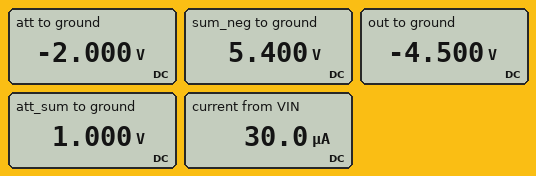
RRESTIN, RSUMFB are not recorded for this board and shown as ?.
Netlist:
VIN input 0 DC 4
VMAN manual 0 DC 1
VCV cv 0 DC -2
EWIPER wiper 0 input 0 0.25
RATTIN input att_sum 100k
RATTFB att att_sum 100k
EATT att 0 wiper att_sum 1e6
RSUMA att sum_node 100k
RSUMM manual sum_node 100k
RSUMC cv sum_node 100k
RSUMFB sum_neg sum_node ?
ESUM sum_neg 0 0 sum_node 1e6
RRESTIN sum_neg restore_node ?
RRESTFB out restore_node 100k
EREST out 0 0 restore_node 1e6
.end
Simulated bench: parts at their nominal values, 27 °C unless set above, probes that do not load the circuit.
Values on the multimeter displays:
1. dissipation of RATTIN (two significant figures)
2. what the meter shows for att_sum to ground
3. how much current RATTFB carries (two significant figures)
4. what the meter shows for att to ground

90 µW
1.000 V
30 µA
-2.000 V
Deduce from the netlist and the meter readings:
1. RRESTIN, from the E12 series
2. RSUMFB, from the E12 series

120 kΩ
180 kΩ
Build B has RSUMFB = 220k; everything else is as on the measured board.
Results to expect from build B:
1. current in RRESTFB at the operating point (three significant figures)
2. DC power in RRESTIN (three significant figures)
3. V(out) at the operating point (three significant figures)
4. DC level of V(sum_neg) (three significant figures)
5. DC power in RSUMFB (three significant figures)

55.0 µA
363 µW
-5.50 V
6.60 V
198 µW
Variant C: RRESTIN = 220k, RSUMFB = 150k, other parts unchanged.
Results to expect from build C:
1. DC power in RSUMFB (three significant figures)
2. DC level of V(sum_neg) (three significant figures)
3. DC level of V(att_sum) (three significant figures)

135 µW
4.50 V
1.00 V
